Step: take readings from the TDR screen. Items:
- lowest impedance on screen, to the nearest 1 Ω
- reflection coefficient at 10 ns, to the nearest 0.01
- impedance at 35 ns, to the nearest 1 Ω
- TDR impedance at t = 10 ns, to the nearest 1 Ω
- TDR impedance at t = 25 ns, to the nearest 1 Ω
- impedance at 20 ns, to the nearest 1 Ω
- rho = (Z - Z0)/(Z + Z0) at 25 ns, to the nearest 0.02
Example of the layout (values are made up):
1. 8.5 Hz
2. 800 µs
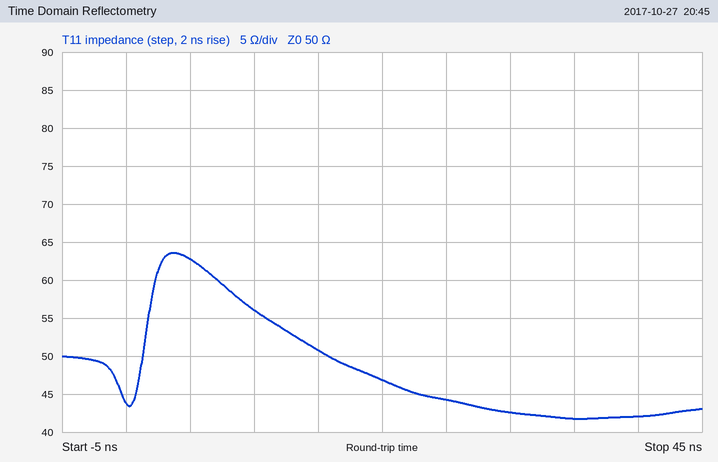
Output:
1. 42 Ω
2. +0.06
3. 42 Ω
4. 56 Ω
5. 44 Ω
6. 47 Ω
7. -0.06
